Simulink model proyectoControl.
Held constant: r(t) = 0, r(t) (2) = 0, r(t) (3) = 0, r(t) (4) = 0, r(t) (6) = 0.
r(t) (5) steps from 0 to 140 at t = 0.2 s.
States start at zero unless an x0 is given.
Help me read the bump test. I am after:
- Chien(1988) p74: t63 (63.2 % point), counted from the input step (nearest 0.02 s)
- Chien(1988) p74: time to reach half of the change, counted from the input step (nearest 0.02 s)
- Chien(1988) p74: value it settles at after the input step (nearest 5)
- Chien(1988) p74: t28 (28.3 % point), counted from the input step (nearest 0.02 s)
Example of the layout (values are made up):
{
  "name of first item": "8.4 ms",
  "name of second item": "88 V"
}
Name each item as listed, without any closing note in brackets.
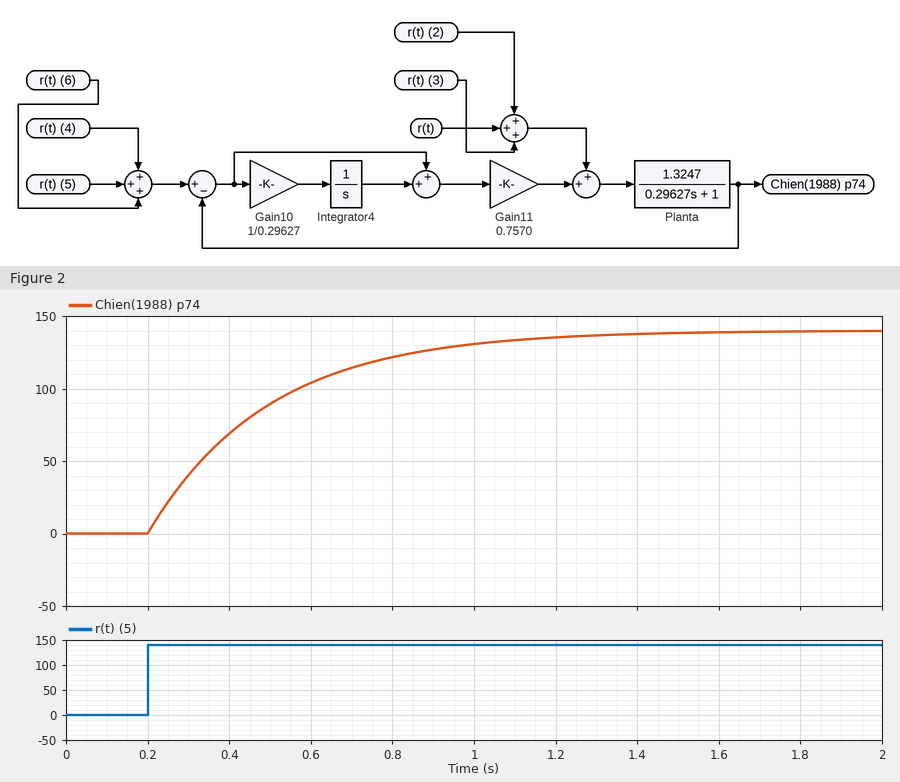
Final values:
{
  "Chien(1988) p74: t63 (63.2 % point), counted from the input step": "0.30 s",
  "Chien(1988) p74: time to reach half of the change, counted from the input step": "0.20 s",
  "Chien(1988) p74: value it settles at after the input step": "140",
  "Chien(1988) p74: t28 (28.3 % point), counted from the input step": "0.10 s"
}
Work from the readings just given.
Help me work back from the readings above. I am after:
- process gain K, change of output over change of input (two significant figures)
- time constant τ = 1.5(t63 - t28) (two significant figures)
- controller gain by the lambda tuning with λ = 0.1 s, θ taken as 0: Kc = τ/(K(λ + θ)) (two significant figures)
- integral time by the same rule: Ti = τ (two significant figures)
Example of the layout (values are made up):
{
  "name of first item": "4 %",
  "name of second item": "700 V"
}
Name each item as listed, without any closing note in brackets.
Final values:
{
  "process gain K, change of output over change of input": "1.0",
  "time constant τ = 1.5(t63 - t28)": "0.30 s",
  "controller gain by the lambda tuning with λ = 0.1 s, θ taken as 0: Kc = τ/(K(λ + θ))": "3.0",
  "integral time by the same rule: Ti = τ": "0.30 s"
}
